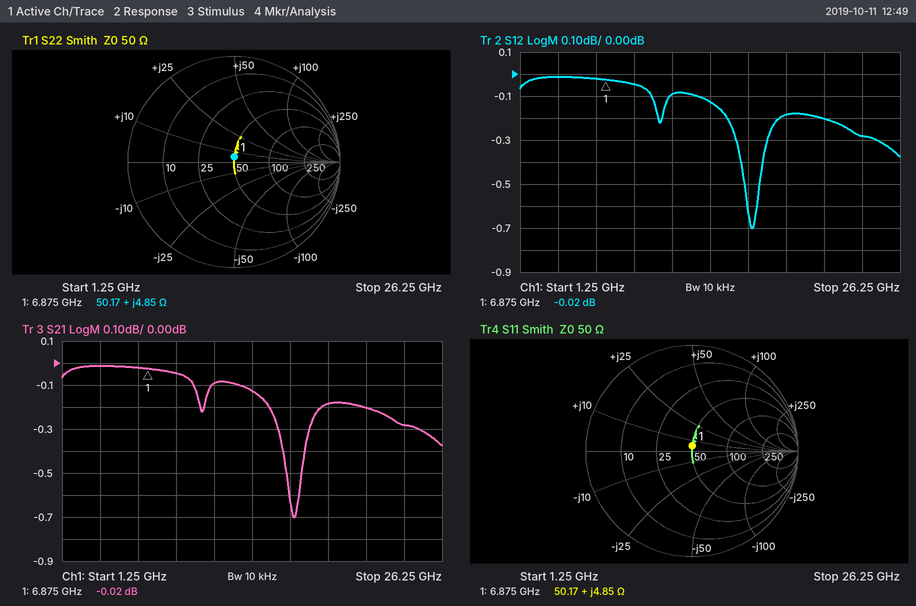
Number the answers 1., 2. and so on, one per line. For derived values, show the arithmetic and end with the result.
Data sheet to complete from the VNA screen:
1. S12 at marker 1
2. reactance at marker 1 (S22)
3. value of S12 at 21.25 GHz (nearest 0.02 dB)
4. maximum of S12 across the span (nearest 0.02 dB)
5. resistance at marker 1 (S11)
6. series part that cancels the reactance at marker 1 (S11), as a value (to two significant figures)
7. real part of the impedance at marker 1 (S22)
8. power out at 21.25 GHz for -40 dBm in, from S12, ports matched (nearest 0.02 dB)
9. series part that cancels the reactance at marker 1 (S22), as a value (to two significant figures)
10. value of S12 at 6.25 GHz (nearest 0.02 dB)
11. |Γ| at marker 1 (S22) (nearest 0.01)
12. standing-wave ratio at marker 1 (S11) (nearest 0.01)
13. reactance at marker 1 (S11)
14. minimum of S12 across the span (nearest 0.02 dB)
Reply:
1. -0.02 dB
2. +4.85 Ω
3. -0.20 dB
4. -0.02 dB
5. 50.17 Ω
6. C = 1/(2π × 6.875 GHz × 4.85 Ω) ≈ 4.8 pF
7. 50.17 Ω
8. -40 dBm + (-0.20 dB) = -40.20 dBm
9. C = 1/(2π × 6.875 GHz × 4.85 Ω) ≈ 4.8 pF
10. -0.02 dB
11. 0.05
12. 1.10
13. +4.85 Ω
14. -0.70 dB
